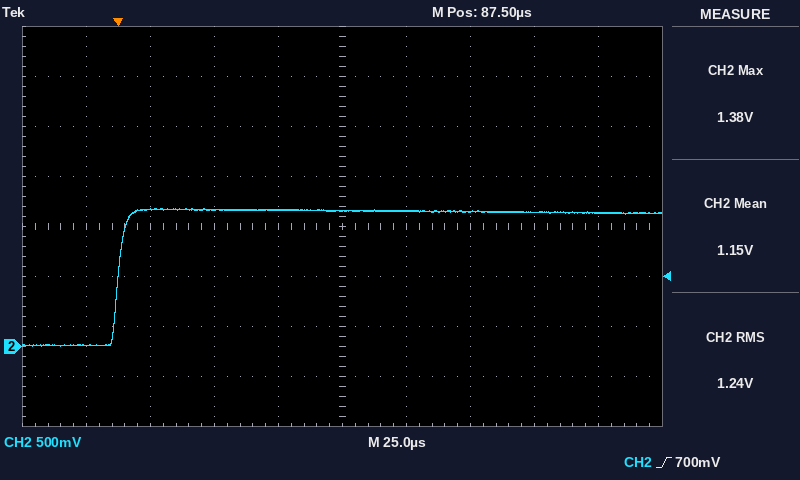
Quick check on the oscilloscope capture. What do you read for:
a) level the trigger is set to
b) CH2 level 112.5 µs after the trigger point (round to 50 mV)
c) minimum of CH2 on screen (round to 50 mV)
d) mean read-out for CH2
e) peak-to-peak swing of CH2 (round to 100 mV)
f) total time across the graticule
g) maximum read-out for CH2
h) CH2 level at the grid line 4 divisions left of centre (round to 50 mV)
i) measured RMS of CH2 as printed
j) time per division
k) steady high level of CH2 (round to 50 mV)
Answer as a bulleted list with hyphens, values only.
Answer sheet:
- 700 mV
- 1.35 V
- 0 mV
- 1.15 V
- 1.40 V
- 250 µs
- 1.38 V
- 0 mV
- 1.24 V
- 25 µs
- 1.35 V
